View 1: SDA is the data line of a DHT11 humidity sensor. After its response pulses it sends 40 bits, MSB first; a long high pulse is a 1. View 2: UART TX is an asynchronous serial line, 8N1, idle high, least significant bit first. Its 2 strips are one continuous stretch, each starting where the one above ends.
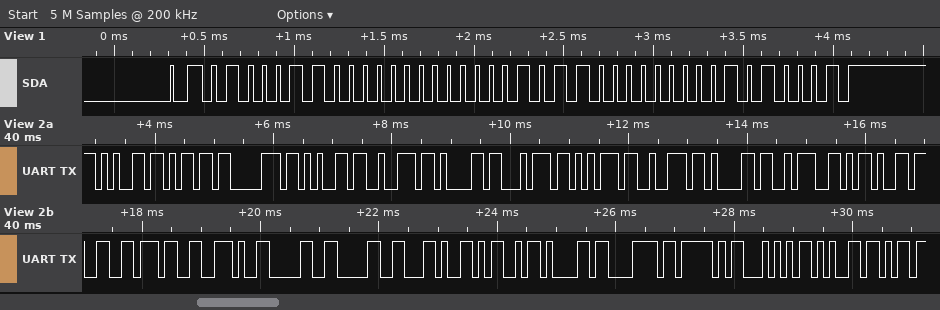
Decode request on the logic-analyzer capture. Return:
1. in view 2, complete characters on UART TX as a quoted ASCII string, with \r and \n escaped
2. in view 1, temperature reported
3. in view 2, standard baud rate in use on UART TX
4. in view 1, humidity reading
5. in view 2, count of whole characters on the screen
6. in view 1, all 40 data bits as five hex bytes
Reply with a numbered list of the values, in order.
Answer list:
1. "emperatura:-37.00,Max_Te"
2. 11.0 °C
3. 9600 baud
4. 70 %
5. 24
6. 46 00 0B 00 51
